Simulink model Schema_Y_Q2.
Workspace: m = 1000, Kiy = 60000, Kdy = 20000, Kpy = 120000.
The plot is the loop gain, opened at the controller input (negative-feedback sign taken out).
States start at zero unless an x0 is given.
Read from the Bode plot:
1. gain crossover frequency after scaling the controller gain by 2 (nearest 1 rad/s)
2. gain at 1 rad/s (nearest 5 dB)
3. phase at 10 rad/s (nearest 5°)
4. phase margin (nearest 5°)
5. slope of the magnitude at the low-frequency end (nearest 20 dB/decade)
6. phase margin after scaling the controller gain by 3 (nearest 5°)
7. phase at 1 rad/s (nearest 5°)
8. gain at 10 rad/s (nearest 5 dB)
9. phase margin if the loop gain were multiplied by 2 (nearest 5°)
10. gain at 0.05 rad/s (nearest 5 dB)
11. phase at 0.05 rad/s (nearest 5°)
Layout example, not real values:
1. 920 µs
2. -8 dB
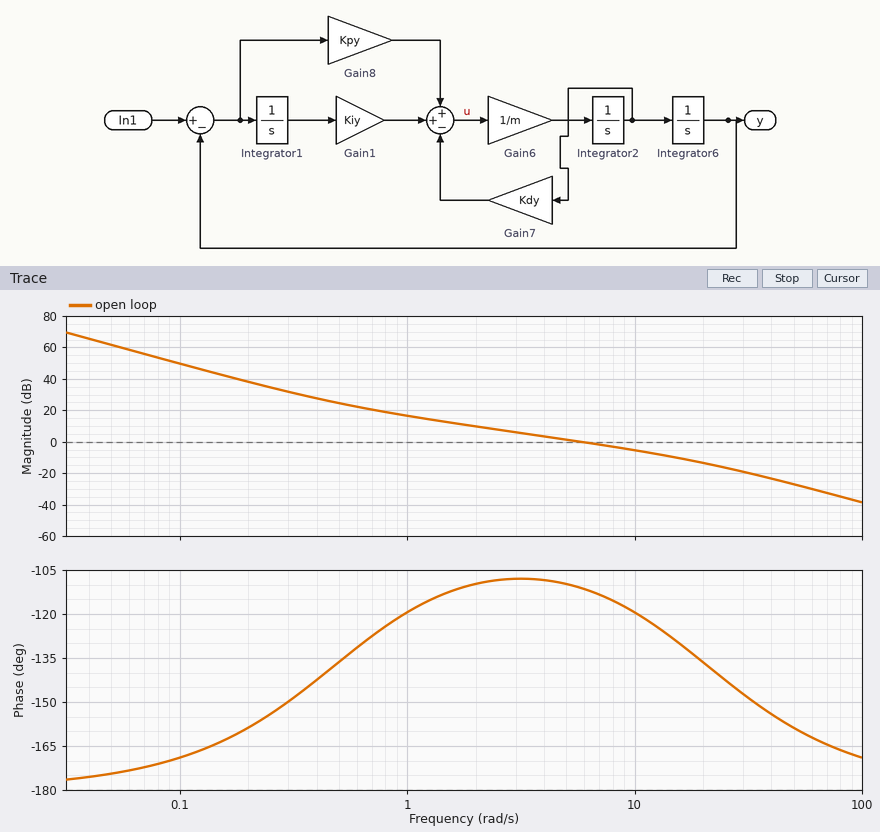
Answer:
1. 11 rad/s
2. 15 dB
3. -120°
4. 70°
5. -40 dB/decade
6. 50°
7. -120°
8. -5 dB
9. 60°
10. 60 dB
11. -175°
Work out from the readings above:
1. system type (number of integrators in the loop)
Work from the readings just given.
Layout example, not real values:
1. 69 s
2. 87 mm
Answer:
1. 2
